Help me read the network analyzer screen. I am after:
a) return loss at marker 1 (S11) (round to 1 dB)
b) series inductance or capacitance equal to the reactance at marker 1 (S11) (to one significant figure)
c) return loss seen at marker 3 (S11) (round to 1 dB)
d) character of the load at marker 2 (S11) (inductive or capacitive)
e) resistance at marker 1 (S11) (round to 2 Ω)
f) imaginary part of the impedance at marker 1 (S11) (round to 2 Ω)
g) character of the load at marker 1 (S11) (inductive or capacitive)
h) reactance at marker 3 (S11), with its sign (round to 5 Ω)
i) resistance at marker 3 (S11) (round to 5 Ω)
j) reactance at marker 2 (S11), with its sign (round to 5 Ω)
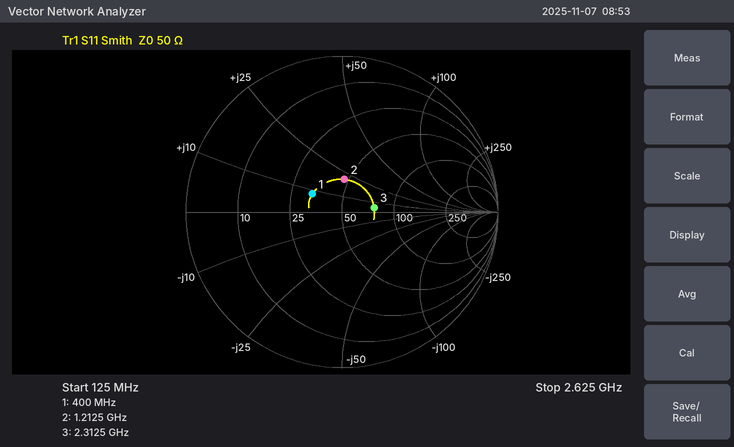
13 dB
3 nH
14 dB
inductive
34 Ω
+8 Ω
inductive
+5 Ω
75 Ω
+20 Ω
